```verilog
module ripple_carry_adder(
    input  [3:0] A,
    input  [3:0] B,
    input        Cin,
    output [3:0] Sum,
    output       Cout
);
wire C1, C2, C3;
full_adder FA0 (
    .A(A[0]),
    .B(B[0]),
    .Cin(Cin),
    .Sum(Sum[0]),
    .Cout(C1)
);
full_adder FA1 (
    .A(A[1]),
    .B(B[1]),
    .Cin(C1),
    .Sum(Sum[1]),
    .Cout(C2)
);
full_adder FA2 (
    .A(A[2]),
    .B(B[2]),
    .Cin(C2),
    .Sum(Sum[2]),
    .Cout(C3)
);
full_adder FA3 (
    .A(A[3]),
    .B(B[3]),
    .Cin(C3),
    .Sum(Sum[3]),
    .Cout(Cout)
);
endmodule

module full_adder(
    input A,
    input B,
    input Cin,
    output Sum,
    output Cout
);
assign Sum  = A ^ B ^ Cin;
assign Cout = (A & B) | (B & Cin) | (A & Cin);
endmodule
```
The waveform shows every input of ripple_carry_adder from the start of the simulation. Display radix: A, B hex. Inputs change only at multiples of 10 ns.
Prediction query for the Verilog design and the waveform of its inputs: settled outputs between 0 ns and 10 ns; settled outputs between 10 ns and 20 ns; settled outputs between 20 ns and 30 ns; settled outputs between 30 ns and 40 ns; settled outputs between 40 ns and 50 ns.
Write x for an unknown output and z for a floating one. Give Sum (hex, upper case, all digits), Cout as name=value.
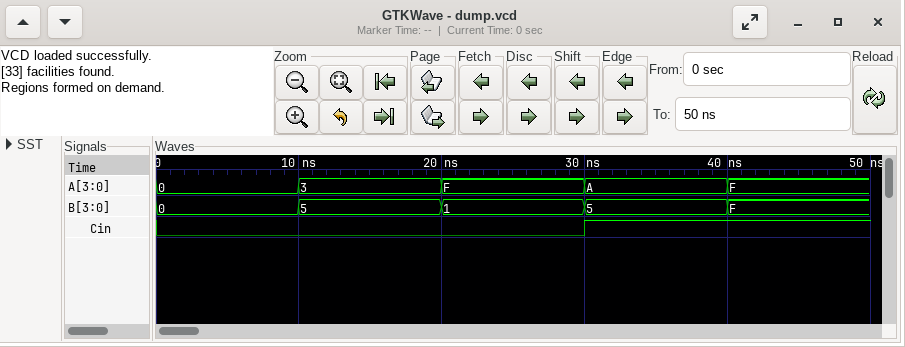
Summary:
Sum=0, Cout=0
Sum=8, Cout=0
Sum=0, Cout=1
Sum=0, Cout=1
Sum=F, Cout=1
